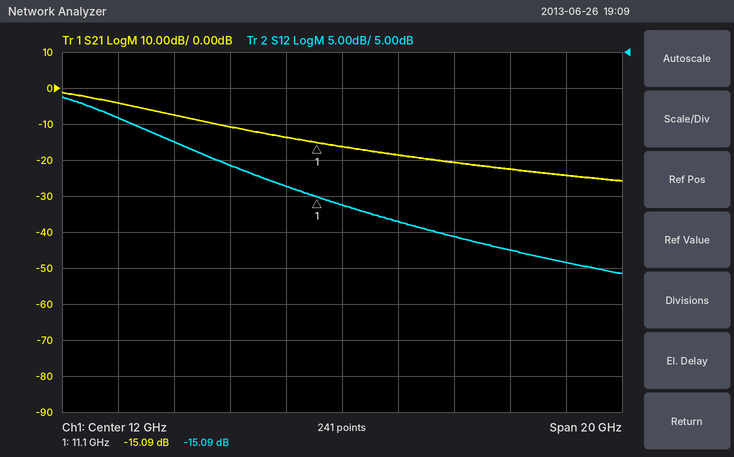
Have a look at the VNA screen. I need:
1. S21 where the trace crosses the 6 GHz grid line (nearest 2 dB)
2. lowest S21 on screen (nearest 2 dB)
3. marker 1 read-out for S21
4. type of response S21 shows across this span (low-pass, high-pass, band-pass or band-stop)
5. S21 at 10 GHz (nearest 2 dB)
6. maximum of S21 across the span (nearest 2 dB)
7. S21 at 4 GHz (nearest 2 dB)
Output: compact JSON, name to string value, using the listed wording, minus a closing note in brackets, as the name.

{"S21 where the trace crosses the 6 GHz grid line": "-8 dB", "lowest S21 on screen": "-26 dB", "marker 1 read-out for S21": "-15.09 dB", "type of response S21 shows across this span": "low-pass", "S21 at 10 GHz": "-14 dB", "maximum of S21 across the span": "-2 dB", "S21 at 4 GHz": "-4 dB"}
